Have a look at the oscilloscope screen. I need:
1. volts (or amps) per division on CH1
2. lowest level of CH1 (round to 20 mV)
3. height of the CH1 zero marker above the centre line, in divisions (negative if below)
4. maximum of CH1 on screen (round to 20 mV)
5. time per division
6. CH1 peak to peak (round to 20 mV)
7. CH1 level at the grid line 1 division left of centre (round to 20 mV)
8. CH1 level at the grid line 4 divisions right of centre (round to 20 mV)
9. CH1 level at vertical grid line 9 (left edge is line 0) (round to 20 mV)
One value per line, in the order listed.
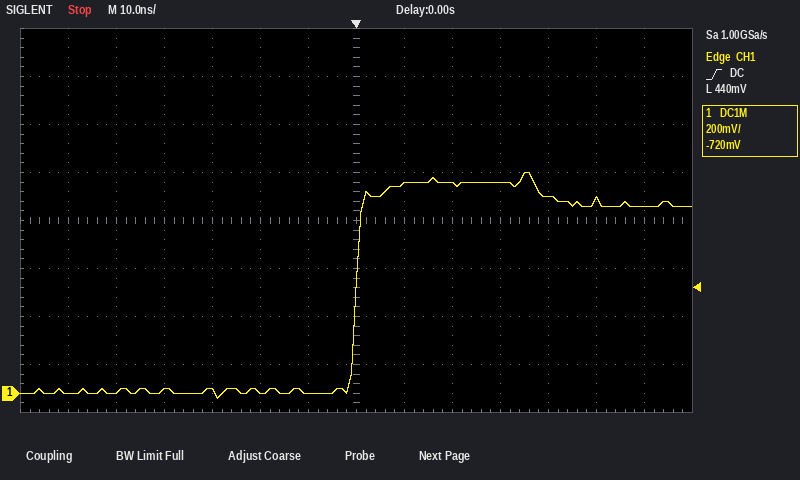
200 mV
-20 mV
-3.6 div
920 mV
10 ns
940 mV
0 mV
820 mV
880 mV
